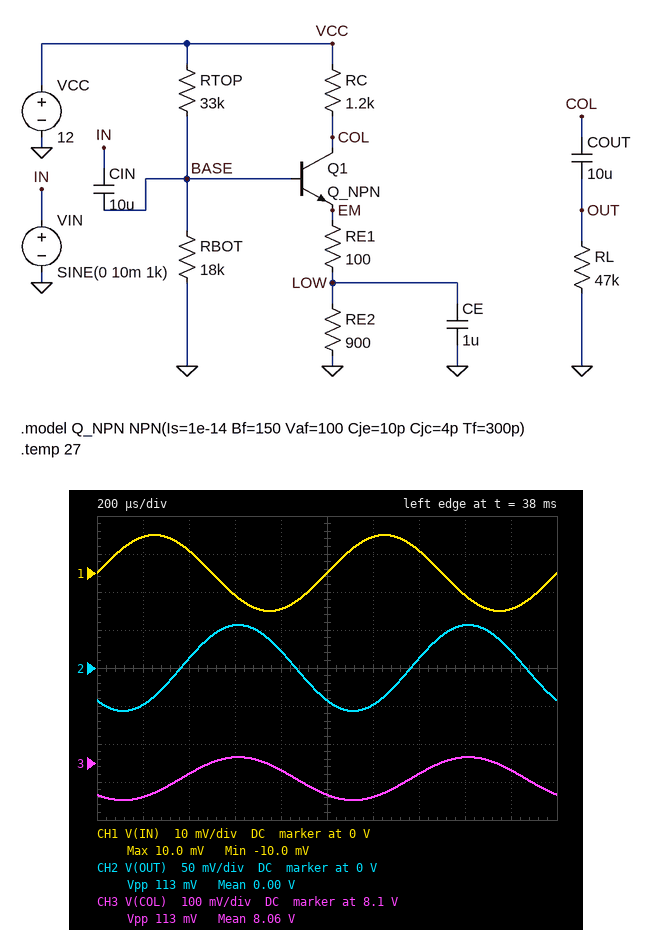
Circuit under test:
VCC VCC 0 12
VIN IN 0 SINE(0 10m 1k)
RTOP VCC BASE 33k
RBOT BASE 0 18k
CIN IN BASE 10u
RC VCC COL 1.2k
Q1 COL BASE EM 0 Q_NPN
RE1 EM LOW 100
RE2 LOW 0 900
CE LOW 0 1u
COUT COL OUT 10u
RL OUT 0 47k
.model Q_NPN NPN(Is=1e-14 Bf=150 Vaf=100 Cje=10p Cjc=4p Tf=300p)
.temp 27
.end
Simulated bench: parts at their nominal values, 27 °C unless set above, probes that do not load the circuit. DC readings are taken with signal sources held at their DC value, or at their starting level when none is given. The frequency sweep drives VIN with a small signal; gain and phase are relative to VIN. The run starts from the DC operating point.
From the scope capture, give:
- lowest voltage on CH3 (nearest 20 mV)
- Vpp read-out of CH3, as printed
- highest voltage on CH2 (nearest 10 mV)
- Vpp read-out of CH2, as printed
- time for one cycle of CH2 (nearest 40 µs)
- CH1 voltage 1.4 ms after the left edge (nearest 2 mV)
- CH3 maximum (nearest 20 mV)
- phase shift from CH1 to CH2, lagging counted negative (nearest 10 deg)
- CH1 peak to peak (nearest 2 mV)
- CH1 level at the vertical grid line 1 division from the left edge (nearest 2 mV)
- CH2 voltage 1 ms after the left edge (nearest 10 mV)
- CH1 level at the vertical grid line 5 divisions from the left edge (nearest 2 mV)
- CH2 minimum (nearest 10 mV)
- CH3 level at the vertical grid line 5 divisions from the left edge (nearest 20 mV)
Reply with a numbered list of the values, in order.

1. 8.00 V
2. 113 mV
3. 60 mV
4. 113 mV
5. 1.00 ms
6. 6 mV
7. 8.12 V
8. -130 deg
9. 20 mV
10. 10 mV
11. -40 mV
12. 0 V
13. -60 mV
14. 8.02 V
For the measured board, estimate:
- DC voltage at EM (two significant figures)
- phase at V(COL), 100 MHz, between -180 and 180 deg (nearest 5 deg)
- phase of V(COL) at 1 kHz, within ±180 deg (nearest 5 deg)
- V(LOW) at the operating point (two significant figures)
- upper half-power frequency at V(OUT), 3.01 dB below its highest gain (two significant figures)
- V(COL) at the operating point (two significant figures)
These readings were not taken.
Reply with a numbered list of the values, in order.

1. 3.3 V
2. 100 deg
3. -130 deg
4. 3.0 V
5. 64 MHz
6. 8.1 V
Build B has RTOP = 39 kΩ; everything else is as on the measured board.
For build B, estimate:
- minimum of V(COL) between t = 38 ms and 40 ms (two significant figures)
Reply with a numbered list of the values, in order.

1. 8.5 V
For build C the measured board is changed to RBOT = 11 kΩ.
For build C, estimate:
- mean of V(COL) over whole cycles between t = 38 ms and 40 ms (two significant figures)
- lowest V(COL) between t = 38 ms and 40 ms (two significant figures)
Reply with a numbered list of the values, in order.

1. 9.4 V
2. 9.3 V
